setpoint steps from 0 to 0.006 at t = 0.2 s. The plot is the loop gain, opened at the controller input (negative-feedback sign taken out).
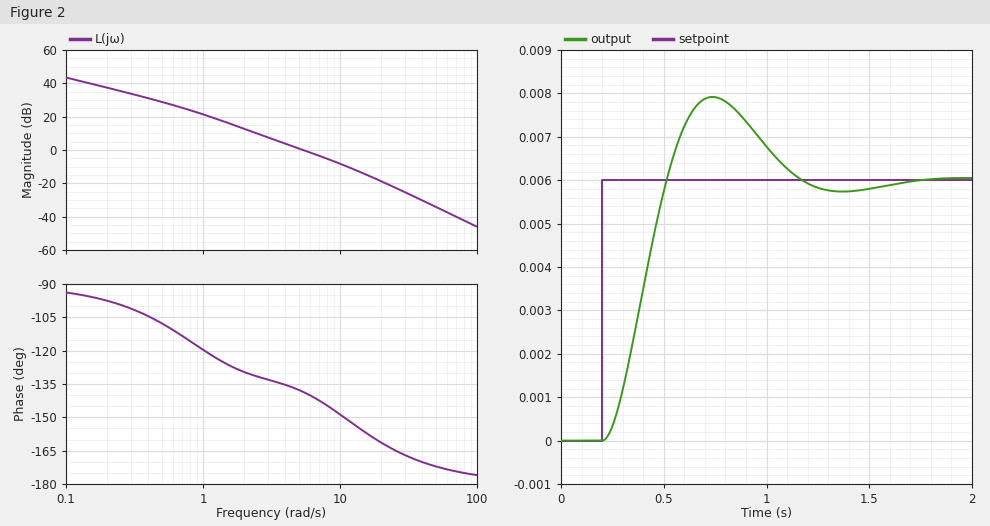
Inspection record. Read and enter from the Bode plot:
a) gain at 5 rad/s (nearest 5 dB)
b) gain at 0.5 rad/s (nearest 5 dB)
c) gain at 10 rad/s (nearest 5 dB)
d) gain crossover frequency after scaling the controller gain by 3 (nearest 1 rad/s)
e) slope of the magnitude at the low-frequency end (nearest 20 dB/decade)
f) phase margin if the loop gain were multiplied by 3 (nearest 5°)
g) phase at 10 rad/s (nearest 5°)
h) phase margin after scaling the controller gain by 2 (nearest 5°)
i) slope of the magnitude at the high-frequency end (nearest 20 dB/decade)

0 dB
30 dB
-10 dB
11 rad/s
-20 dB/decade
30°
-150°
35°
-40 dB/decade
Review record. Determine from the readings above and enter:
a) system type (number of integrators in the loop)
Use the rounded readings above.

1
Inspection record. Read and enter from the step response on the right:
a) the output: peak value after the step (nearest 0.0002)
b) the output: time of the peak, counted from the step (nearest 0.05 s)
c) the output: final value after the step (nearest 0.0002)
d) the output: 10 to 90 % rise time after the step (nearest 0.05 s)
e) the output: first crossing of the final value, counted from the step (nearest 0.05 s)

0.0080
0.55 s
0.0060
0.20 s
0.30 s
